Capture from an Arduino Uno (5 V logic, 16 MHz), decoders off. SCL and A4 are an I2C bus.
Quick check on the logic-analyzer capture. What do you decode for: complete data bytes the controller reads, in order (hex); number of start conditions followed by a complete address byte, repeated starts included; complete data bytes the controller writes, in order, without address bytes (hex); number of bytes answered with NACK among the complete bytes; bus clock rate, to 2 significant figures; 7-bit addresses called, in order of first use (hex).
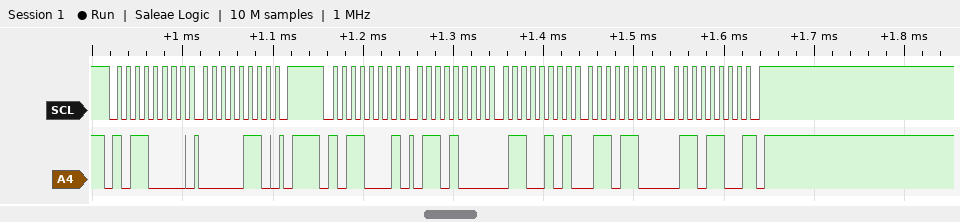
68 65 6C 6C
2
06
1
100 kHz
0x58
